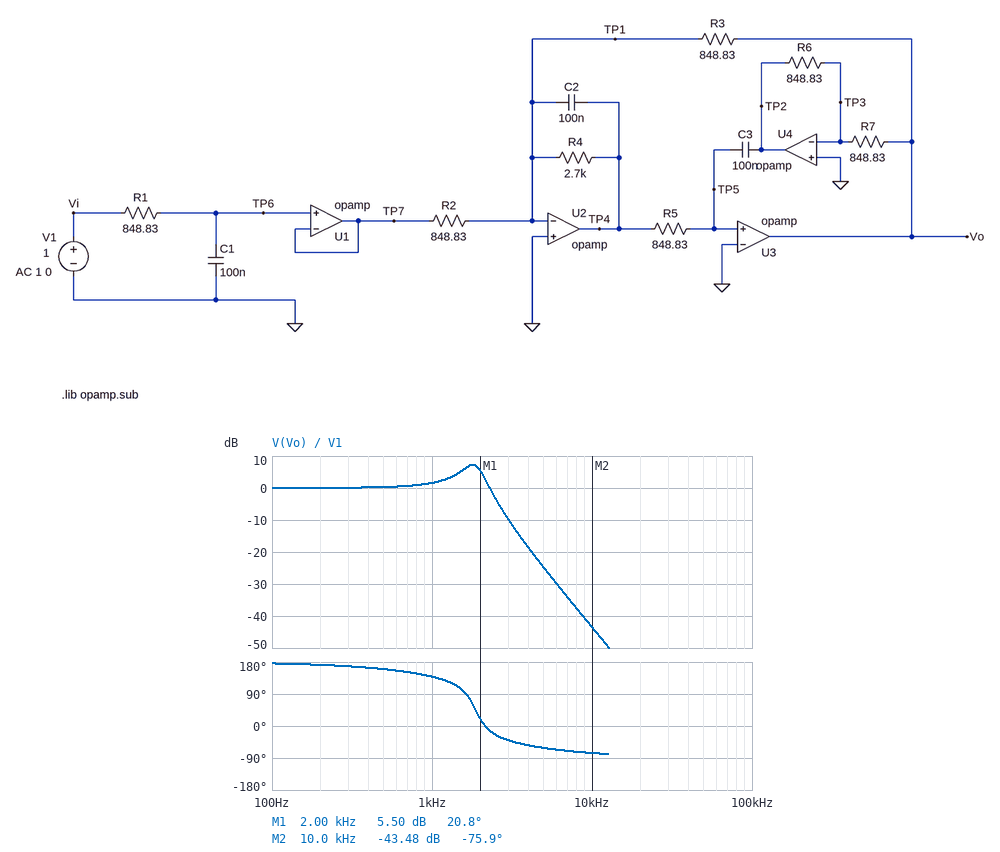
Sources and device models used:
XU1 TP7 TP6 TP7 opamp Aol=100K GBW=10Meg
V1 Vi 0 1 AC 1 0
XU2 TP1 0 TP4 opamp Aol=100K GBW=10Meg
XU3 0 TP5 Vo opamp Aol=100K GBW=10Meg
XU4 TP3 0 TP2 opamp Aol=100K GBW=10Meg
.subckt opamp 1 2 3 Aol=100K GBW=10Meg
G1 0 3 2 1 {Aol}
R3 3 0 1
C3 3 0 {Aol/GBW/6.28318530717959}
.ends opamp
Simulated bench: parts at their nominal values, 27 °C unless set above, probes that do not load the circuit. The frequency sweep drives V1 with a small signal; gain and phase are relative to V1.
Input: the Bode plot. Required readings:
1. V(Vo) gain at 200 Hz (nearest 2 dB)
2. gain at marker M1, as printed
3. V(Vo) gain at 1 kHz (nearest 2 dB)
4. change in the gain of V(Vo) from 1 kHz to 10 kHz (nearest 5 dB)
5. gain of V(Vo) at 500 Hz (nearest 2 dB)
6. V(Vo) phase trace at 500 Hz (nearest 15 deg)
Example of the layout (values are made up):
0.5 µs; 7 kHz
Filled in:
0 dB; 5.50 dB; 2 dB; -45 dB; 0 dB; 165 deg
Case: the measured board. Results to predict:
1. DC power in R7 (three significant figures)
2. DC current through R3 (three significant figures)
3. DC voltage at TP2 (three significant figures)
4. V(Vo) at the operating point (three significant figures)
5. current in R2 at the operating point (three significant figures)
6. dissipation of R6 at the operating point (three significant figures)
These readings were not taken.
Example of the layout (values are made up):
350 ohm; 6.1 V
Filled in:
1.18 mW; 1.18 mA; 1.00 V; -1.00 V; 1.18 mA; 1.18 mW
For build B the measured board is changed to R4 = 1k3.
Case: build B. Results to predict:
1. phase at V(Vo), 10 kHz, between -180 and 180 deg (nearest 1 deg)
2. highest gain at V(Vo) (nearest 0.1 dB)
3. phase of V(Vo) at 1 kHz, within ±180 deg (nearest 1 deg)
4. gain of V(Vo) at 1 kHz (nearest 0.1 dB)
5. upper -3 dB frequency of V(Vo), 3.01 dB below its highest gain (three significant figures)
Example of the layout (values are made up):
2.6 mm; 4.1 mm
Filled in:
-72 deg; 1.8 dB; 126 deg; 0.9 dB; 2.09 kHz
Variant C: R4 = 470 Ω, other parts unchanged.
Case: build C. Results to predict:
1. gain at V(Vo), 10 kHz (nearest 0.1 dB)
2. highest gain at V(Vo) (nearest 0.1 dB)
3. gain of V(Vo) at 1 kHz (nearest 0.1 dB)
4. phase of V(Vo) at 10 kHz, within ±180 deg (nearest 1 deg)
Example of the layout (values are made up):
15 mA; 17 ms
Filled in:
-44.0 dB; 0 dB; -2.7 dB; -60 deg
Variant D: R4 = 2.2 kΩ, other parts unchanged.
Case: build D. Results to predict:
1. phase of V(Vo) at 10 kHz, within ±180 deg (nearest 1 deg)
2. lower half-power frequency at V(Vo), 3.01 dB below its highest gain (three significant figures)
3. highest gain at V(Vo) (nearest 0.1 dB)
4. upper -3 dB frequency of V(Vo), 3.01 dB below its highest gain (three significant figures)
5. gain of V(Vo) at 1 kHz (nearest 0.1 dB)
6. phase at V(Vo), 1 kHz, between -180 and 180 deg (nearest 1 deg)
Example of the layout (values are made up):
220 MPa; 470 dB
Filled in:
-75 deg; 1.24 kHz; 5.6 dB; 2.09 kHz; 1.5 dB; 136 deg
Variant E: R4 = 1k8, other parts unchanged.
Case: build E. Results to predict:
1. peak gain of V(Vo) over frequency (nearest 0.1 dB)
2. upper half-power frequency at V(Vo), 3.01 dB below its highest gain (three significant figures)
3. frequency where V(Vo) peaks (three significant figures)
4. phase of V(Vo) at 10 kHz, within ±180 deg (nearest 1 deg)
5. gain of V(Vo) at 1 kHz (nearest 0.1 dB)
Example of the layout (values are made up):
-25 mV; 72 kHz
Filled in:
4.1 dB; 2.10 kHz; 1.71 kHz; -74 deg; 1.3 dB
